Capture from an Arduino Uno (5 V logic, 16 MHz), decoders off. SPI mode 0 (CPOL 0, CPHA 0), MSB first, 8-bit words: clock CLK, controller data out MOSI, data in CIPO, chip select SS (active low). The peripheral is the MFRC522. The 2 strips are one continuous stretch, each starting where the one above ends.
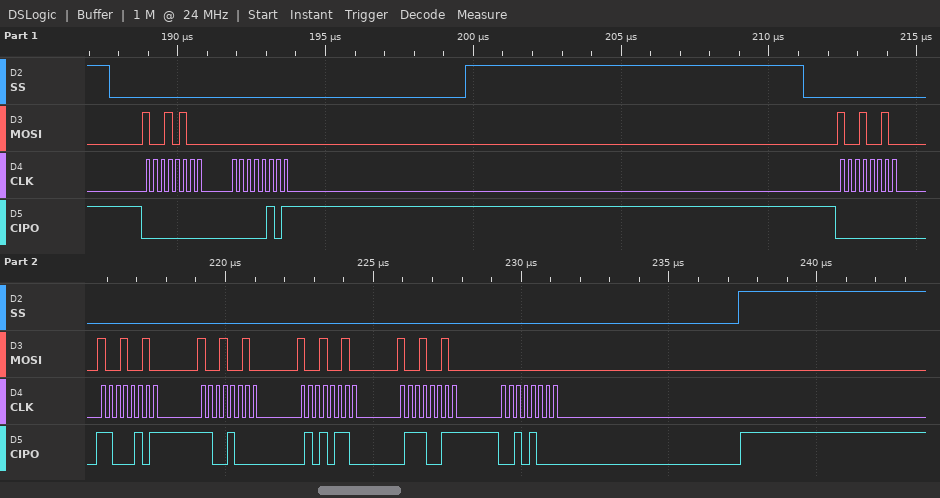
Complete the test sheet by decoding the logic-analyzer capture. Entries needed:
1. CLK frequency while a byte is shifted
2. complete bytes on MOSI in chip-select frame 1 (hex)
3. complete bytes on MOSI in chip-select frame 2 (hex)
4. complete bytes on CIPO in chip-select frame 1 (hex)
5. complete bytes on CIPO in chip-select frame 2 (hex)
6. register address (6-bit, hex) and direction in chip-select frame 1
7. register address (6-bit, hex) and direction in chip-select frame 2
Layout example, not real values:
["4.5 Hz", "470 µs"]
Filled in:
["4 MHz", "94 00", "92 92 92 92 92 00", "00 05", "00 C5 C8 56 73 28", "0x0A read", "0x09 read"]
